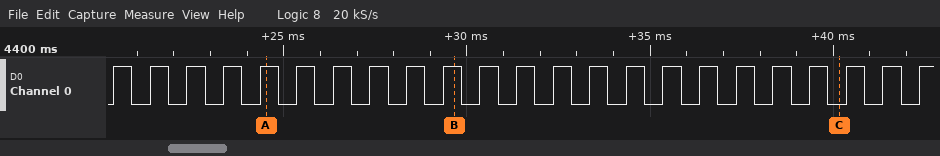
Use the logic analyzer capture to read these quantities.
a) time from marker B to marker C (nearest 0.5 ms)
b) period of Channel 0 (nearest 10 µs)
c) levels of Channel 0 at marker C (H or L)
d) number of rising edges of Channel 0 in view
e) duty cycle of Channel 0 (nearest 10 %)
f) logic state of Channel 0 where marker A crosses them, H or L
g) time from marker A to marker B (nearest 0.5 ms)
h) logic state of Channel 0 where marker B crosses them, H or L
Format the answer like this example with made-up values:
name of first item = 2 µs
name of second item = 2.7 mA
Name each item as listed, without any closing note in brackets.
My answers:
time from marker B to marker C = 10.5 ms
period of Channel 0 = 1000 µs
levels of Channel 0 at marker C = Channel 0=L
number of rising edges of Channel 0 in view = 23
duty cycle of Channel 0 = 50 %
logic state of Channel 0 where marker A crosses them, H or L = Channel 0=H
time from marker A to marker B = 5 ms
logic state of Channel 0 where marker B crosses them, H or L = Channel 0=H
